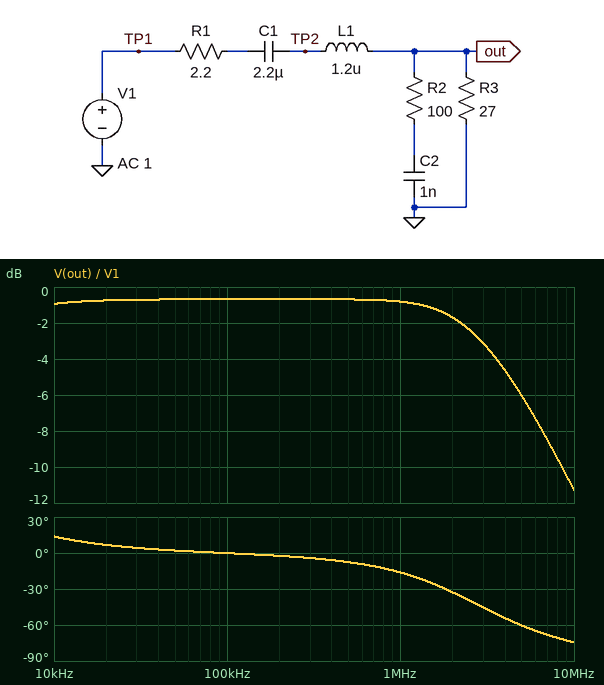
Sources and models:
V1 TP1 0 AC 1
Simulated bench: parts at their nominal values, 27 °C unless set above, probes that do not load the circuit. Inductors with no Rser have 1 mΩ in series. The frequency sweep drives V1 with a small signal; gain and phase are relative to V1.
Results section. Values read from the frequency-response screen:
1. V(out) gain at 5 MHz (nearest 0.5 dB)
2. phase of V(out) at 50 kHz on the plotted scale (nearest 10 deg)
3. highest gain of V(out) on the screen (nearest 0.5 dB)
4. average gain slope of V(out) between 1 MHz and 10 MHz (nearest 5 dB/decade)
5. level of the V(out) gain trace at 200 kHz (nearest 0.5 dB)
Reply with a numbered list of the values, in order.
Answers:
1. -6.0 dB
2. 0 deg
3. -0.5 dB
4. -10 dB/decade
5. -0.5 dB
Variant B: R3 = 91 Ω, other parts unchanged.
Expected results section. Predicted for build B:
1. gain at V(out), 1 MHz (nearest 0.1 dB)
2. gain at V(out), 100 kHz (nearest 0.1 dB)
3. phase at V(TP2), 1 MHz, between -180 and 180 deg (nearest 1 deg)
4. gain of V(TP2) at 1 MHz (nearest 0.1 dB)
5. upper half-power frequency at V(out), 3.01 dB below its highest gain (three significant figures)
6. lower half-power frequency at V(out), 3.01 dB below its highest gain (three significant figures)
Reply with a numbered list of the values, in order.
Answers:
1. 0 dB
2. -0.2 dB
3. 0 deg
4. -0.3 dB
5. 6.82 MHz
6. 822 Hz
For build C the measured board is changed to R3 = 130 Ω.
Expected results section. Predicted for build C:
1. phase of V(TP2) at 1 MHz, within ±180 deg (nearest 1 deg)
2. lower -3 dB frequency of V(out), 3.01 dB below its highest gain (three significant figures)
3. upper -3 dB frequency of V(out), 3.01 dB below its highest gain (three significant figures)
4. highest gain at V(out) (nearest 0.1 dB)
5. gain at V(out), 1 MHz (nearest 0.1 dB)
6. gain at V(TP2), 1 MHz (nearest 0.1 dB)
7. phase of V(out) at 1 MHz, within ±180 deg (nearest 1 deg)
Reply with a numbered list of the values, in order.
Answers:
1. 0 deg
2. 590 Hz
3. 7.91 MHz
4. 0.2 dB
5. 0.1 dB
6. -0.2 dB
7. -5 deg
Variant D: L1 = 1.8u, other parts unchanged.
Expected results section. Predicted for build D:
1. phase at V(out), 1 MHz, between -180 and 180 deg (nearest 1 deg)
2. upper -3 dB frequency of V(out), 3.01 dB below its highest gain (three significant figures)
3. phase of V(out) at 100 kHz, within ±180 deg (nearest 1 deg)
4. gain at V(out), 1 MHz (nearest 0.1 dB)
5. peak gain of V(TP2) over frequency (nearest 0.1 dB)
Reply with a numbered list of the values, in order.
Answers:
1. -24 deg
2. 2.36 MHz
3. -1 deg
4. -1.1 dB
5. 0 dB
